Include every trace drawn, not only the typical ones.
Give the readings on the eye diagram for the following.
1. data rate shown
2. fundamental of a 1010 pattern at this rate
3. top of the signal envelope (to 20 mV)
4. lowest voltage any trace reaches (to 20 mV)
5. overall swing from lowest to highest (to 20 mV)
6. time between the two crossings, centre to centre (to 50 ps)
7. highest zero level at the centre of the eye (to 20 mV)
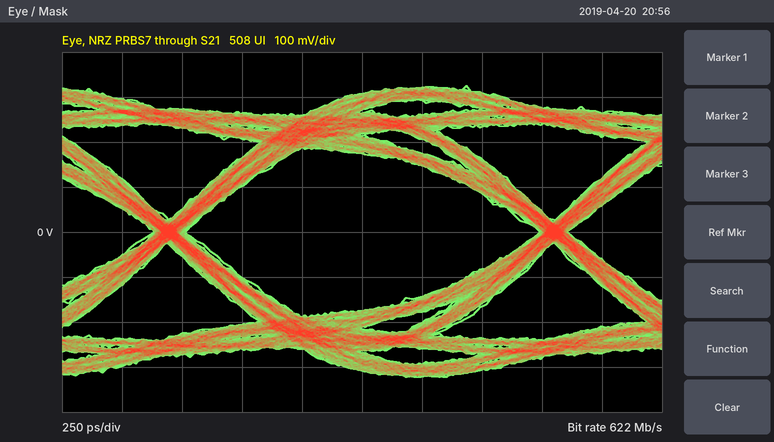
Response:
622 Mb/s
311 MHz
320 mV
-320 mV
640 mV
1.60 ns
-180 mV
